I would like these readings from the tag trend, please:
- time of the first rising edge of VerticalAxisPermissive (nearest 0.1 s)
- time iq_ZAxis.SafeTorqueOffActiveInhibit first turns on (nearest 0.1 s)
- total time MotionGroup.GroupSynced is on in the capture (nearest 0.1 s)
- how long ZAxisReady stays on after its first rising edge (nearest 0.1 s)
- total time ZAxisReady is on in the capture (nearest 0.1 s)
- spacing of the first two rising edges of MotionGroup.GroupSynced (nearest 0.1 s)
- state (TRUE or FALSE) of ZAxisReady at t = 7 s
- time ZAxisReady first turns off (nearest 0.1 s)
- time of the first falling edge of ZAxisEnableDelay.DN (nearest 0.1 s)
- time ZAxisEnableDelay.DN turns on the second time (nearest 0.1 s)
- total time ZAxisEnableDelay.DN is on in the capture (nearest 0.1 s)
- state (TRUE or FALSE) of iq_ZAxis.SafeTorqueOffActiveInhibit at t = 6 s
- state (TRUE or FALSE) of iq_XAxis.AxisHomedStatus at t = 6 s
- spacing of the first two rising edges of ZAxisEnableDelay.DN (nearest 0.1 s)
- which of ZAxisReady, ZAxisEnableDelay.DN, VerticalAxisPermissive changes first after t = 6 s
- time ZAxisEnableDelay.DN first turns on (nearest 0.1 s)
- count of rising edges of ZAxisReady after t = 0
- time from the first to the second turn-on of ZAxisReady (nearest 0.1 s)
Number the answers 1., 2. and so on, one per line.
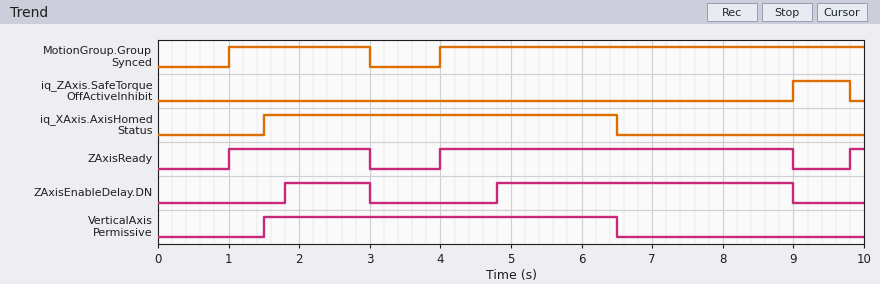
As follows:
1. 1.5 s
2. 9.0 s
3. 8.0 s
4. 2.0 s
5. 7.2 s
6. 3.0 s
7. TRUE
8. 3.0 s
9. 3.0 s
10. 4.8 s
11. 5.4 s
12. FALSE
13. TRUE
14. 3.0 s
15. VerticalAxisPermissive
16. 1.8 s
17. 3
18. 3.0 s
